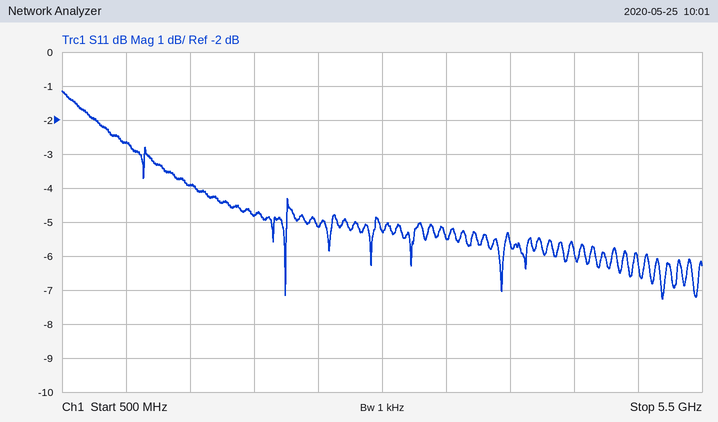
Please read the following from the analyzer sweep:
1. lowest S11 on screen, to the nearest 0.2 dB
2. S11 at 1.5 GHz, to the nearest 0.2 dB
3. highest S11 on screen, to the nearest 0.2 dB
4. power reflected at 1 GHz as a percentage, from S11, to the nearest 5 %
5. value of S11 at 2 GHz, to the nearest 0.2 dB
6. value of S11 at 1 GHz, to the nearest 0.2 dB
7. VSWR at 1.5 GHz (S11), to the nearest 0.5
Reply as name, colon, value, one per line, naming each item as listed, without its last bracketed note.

lowest S11 on screen, to the nearest 0.2 dB: -7.2 dB
S11 at 1.5 GHz, to the nearest 0.2 dB: -4.0 dB
highest S11 on screen, to the nearest 0.2 dB: -1.2 dB
power reflected at 1 GHz as a percentage, from S11, to the nearest 5 %: 55 %
value of S11 at 2 GHz, to the nearest 0.2 dB: -4.8 dB
value of S11 at 1 GHz, to the nearest 0.2 dB: -2.6 dB
VSWR at 1.5 GHz (S11), to the nearest 0.5: 4.5
